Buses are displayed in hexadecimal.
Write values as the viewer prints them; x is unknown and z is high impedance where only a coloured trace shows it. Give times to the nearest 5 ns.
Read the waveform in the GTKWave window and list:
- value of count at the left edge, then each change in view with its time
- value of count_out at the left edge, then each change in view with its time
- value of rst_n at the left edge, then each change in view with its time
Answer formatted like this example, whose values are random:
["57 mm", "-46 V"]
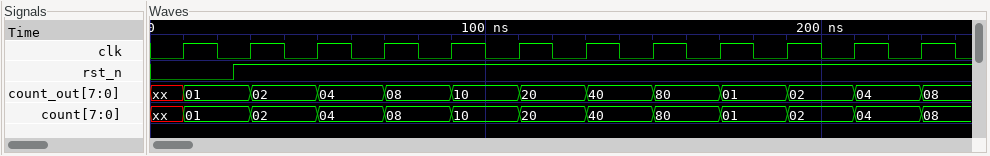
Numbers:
["xx, 01 at 10 ns, 02 at 30 ns, 04 at 50 ns, 08 at 70 ns, 10 at 90 ns, 20 at 110 ns, 40 at 130 ns, 80 at 150 ns, 01 at 170 ns, 02 at 190 ns, 04 at 210 ns, 08 at 230 ns", "xx, 01 at 10 ns, 02 at 30 ns, 04 at 50 ns, 08 at 70 ns, 10 at 90 ns, 20 at 110 ns, 40 at 130 ns, 80 at 150 ns, 01 at 170 ns, 02 at 190 ns, 04 at 210 ns, 08 at 230 ns", "0, 1 at 25 ns"]
